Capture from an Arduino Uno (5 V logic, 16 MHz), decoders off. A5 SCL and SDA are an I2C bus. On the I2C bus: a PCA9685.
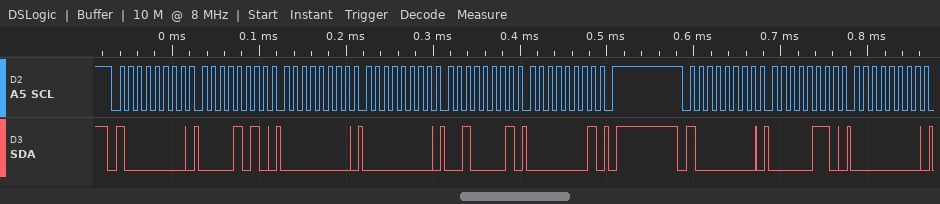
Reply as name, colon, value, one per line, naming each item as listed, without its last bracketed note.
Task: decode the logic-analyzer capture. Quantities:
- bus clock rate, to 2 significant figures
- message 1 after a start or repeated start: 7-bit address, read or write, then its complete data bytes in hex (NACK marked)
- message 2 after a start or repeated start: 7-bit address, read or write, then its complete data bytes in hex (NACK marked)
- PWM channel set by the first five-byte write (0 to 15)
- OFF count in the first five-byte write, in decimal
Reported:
bus clock rate, to 2 significant figures: 100 kHz
message 1 after a start or repeated start: 7-bit address, read or write, then its complete data bytes in hex: 0x40 write: 0A 00 00 21 01
message 2 after a start or repeated start: 7-bit address, read or write, then its complete data bytes in hex: 0x40 write: 06 00
PWM channel set by the first five-byte write: 1
OFF count in the first five-byte write, in decimal: 289
